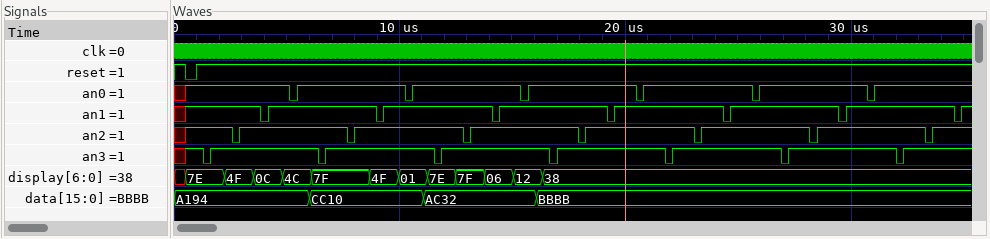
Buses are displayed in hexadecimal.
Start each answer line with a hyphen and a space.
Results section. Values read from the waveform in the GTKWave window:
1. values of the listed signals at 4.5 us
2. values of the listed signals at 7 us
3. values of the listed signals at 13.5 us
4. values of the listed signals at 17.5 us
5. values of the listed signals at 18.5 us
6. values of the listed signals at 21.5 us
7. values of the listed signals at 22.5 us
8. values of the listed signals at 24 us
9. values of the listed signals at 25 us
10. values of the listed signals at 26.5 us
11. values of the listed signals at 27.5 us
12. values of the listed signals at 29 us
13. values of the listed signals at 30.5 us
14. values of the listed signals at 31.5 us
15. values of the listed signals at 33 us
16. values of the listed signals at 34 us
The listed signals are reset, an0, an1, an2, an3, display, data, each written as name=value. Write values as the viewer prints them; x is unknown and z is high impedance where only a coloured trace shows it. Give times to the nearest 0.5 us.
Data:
- reset=1, an0=1, an1=1, an2=1, an3=1, display=0C, data=A194
- reset=1, an0=1, an1=1, an2=1, an3=1, display=7F, data=CC10
- reset=1, an0=1, an1=1, an2=1, an3=1, display=7F, data=AC32
- reset=1, an0=1, an1=1, an2=1, an3=1, display=38, data=BBBB
- reset=1, an0=1, an1=1, an2=1, an3=1, display=38, data=BBBB
- reset=1, an0=1, an1=1, an2=1, an3=1, display=38, data=BBBB
- reset=1, an0=1, an1=1, an2=1, an3=1, display=38, data=BBBB
- reset=1, an0=1, an1=1, an2=1, an3=1, display=38, data=BBBB
- reset=1, an0=1, an1=1, an2=1, an3=1, display=38, data=BBBB
- reset=1, an0=1, an1=1, an2=1, an3=1, display=38, data=BBBB
- reset=1, an0=1, an1=1, an2=1, an3=1, display=38, data=BBBB
- reset=1, an0=1, an1=1, an2=1, an3=1, display=38, data=BBBB
- reset=1, an0=1, an1=1, an2=1, an3=1, display=38, data=BBBB
- reset=1, an0=1, an1=1, an2=1, an3=1, display=38, data=BBBB
- reset=1, an0=1, an1=1, an2=1, an3=1, display=38, data=BBBB
- reset=1, an0=1, an1=1, an2=1, an3=1, display=38, data=BBBB
